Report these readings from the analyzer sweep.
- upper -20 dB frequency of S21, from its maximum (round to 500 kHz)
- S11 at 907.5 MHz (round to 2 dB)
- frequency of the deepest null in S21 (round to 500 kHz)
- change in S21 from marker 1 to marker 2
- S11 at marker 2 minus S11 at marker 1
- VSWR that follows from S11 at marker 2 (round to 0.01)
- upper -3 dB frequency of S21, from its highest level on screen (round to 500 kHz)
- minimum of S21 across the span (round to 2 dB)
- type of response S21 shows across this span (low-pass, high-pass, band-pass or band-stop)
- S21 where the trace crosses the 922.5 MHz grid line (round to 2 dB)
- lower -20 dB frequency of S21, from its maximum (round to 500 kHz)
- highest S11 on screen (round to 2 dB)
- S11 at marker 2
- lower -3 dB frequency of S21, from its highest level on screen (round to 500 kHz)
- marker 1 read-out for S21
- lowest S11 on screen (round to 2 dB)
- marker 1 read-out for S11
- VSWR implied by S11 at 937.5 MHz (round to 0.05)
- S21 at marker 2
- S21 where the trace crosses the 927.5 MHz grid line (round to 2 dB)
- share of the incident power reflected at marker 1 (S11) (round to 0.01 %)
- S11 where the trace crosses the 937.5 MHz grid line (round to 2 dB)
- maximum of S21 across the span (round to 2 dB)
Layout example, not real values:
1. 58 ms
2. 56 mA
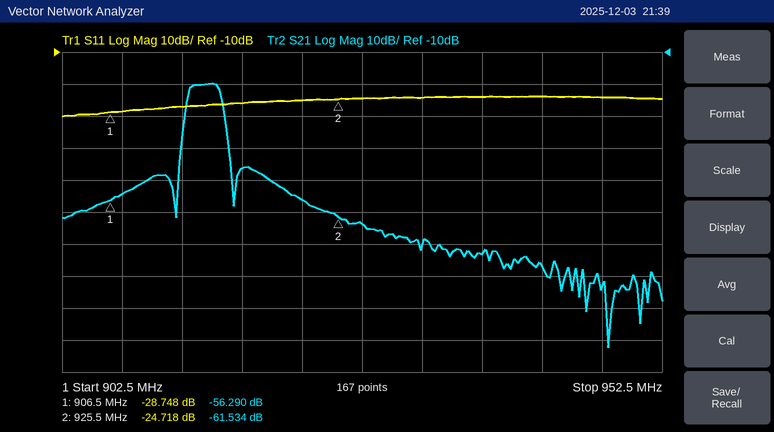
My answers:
1. 916.5 MHz
2. -28 dB
3. 948.0 MHz
4. -5.244 dB
5. 4.030 dB
6. 1.12
7. 915.5 MHz
8. -102 dB
9. band-pass
10. -56 dB
11. 912.5 MHz
12. -24 dB
13. -24.718 dB
14. 913.0 MHz
15. -56.290 dB
16. -30 dB
17. -28.748 dB
18. 1.15
19. -61.534 dB
20. -64 dB
21. 0.13 %
22. -24 dB
23. -20 dB
